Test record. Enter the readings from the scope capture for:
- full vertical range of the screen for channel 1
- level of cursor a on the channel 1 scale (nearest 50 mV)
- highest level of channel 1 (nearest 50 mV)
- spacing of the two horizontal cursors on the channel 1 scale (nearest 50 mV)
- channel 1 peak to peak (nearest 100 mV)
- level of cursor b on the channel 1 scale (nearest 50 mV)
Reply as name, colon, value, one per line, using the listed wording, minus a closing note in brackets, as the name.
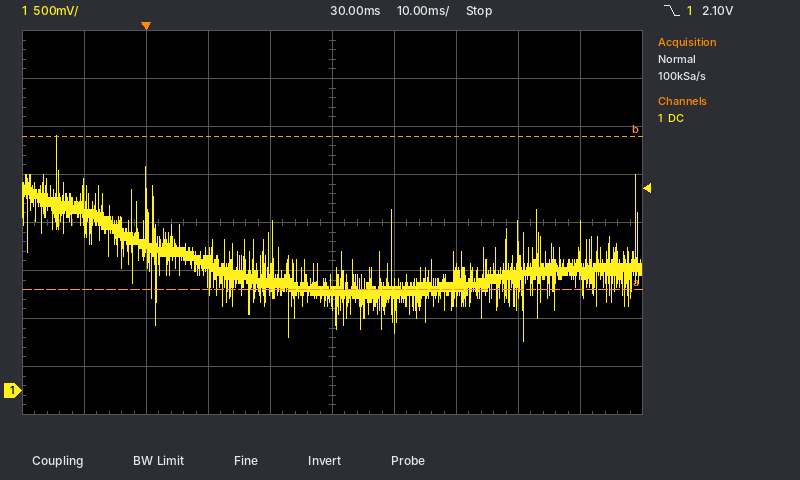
full vertical range of the screen for channel 1: 4 V
level of cursor a on the channel 1 scale: 1.05 V
highest level of channel 1: 2.65 V
spacing of the two horizontal cursors on the channel 1 scale: 1.60 V
channel 1 peak to peak: 2.10 V
level of cursor b on the channel 1 scale: 2.65 V
